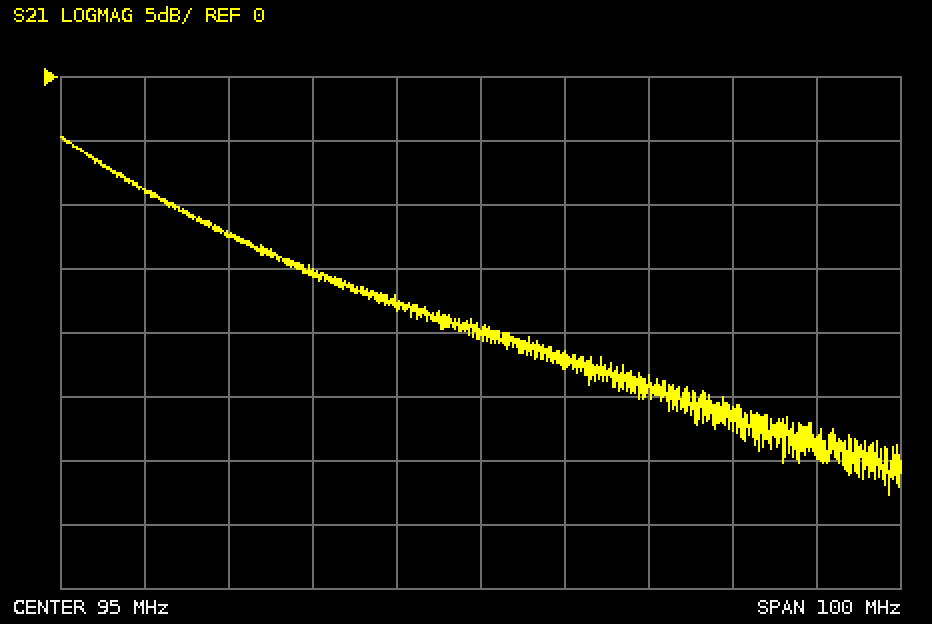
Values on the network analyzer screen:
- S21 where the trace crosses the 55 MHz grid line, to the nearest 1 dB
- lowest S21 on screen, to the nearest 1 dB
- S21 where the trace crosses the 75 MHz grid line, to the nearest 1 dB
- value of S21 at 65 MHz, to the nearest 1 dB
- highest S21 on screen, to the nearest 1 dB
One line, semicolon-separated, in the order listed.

-9 dB; -33 dB; -15 dB; -12 dB; -5 dB
